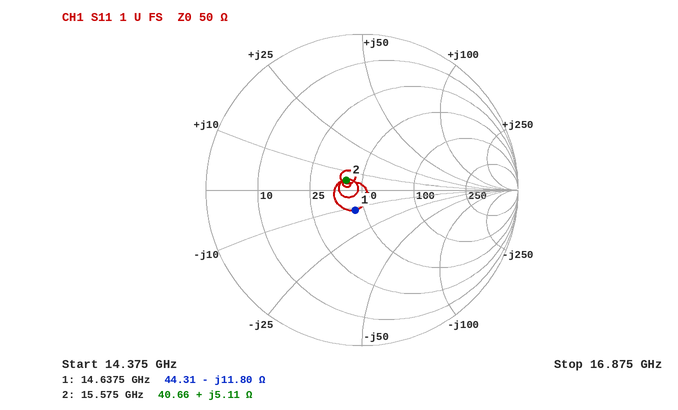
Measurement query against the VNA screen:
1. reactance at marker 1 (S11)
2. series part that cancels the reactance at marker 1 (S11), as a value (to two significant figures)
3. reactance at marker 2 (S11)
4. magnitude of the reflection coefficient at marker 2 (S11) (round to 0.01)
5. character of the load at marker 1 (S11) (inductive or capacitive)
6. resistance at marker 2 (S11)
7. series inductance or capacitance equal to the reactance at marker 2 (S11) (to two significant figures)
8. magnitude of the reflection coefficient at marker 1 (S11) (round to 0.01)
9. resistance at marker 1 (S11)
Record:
-11.80 Ω
130 pH
+5.11 Ω
0.12
capacitive
40.66 Ω
52 pH
0.14
44.31 Ω
